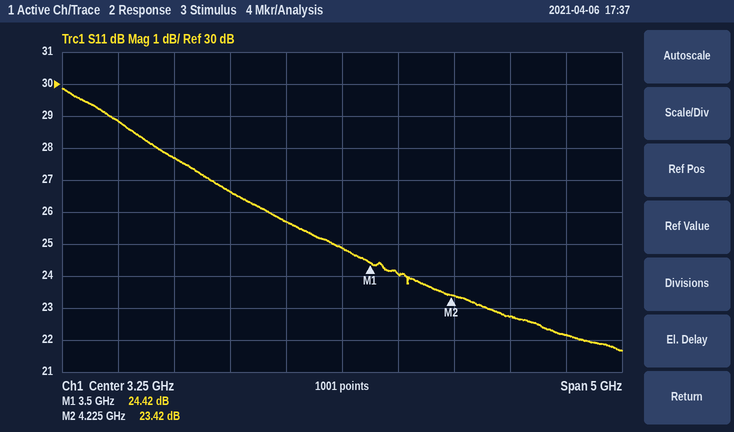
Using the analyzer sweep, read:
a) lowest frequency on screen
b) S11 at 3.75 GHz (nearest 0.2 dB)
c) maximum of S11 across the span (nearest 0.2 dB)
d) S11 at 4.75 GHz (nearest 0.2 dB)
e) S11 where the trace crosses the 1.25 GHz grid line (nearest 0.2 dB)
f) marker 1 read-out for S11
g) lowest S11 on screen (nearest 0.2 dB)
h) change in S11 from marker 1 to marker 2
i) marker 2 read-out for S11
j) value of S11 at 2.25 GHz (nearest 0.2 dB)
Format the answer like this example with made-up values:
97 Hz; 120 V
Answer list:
750 MHz; 24.0 dB; 29.8 dB; 22.8 dB; 28.8 dB; 24.42 dB; 21.6 dB; -1.00 dB; 23.42 dB; 26.6 dB
